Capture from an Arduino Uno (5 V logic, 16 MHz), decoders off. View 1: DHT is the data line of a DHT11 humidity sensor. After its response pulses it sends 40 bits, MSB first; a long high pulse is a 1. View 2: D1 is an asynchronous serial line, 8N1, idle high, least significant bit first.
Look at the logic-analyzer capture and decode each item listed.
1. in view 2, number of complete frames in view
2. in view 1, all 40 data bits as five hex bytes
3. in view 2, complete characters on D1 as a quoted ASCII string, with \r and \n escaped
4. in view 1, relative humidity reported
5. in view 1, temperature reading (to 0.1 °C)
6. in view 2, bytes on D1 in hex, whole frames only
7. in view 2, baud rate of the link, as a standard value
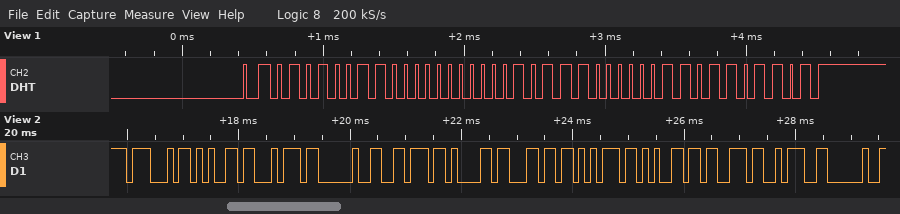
12
53 00 17 03 6D
"Get values: "
83 %
23.3 °C
47 65 74 20 76 61 6C 75 65 73 3A 20
9600 baud
